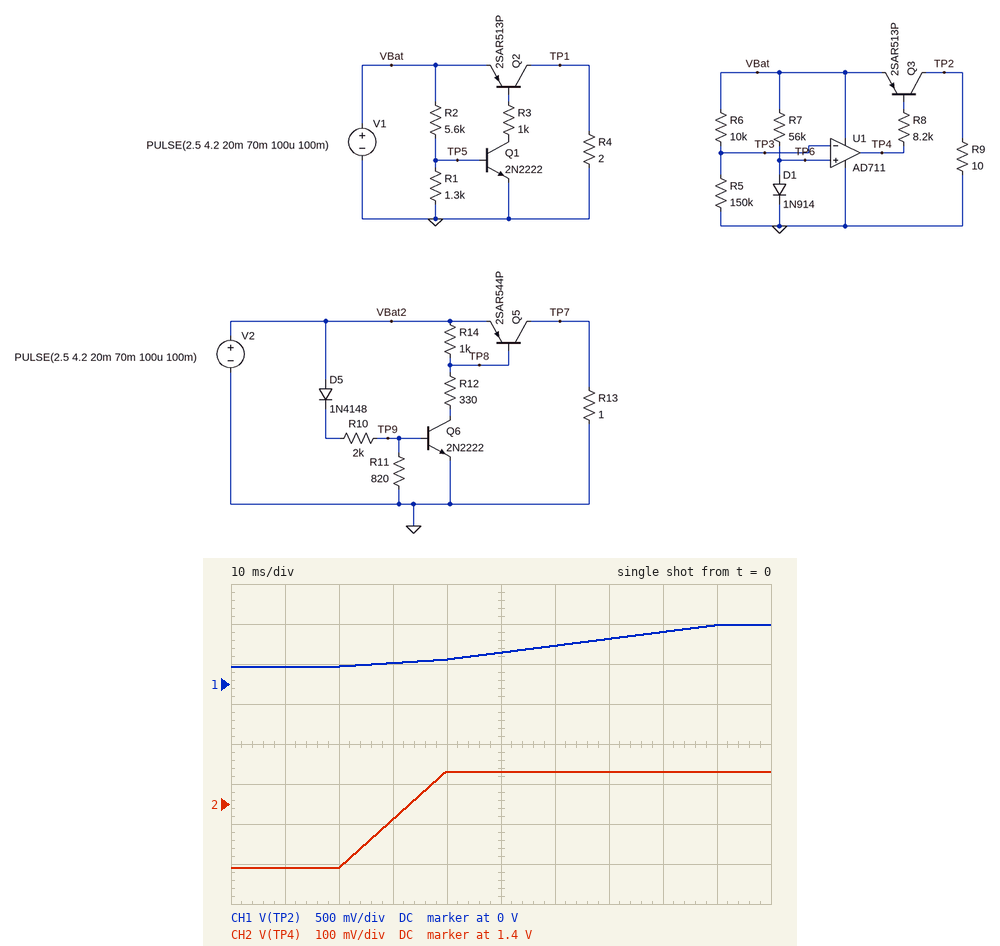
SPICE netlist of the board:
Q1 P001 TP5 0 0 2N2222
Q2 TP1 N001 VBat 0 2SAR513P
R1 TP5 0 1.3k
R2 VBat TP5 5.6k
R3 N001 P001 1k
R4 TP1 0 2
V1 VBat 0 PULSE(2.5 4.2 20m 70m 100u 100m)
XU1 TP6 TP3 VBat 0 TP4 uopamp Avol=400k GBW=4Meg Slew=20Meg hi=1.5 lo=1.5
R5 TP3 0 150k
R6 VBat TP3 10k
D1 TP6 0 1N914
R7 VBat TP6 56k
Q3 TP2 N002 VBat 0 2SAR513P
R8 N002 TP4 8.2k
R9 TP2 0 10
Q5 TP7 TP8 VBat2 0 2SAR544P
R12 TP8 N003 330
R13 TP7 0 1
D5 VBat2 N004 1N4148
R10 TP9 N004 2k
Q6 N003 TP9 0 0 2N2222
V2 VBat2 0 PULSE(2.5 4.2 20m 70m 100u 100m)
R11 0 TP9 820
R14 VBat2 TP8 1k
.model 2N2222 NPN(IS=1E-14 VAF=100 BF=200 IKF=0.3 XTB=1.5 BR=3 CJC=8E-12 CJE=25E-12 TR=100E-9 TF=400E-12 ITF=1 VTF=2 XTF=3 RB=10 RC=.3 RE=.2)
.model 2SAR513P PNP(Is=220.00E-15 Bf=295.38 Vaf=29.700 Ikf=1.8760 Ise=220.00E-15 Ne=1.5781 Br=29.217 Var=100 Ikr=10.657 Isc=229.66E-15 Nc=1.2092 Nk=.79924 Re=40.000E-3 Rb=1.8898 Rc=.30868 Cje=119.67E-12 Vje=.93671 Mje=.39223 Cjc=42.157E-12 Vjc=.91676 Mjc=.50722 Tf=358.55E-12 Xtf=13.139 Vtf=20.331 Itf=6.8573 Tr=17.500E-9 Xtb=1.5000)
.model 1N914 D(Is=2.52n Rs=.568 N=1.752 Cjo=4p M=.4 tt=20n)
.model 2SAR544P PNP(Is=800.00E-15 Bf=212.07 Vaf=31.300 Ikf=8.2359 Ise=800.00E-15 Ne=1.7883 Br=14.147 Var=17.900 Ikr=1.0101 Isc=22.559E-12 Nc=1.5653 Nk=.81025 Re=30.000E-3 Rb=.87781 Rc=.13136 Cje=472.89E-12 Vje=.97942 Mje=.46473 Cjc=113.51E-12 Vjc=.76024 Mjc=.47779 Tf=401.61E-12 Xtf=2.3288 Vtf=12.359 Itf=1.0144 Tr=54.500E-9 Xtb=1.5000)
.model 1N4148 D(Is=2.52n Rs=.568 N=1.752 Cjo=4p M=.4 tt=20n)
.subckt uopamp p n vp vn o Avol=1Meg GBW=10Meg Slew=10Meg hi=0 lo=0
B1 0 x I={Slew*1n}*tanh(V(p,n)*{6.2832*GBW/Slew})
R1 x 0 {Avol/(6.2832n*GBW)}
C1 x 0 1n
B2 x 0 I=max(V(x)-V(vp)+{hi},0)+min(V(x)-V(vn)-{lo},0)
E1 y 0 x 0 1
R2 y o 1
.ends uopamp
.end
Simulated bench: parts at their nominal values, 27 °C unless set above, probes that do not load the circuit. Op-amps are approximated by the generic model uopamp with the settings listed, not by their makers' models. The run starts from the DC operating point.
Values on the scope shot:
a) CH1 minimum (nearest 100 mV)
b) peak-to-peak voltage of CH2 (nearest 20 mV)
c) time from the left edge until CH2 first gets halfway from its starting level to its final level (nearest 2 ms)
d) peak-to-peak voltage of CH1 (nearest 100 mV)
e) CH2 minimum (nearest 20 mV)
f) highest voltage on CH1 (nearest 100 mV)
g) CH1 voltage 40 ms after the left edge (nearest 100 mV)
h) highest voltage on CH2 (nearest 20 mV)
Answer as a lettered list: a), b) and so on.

a) 200 mV
b) 240 mV
c) 30 ms
d) 500 mV
e) 1.24 V
f) 700 mV
g) 300 mV
h) 1.48 V
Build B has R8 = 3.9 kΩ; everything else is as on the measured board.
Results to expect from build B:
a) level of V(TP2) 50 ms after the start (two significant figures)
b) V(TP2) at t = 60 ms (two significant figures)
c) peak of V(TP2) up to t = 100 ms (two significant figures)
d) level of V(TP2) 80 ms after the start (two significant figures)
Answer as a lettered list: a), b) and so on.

a) 780 mV
b) 940 mV
c) 1.4 V
d) 1.3 V
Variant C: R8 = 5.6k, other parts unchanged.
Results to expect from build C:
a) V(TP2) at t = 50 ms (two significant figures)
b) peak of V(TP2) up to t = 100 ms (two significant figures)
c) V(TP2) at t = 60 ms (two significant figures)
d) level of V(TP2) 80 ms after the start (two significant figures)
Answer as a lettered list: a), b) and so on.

a) 560 mV
b) 1.0 V
c) 680 mV
d) 920 mV
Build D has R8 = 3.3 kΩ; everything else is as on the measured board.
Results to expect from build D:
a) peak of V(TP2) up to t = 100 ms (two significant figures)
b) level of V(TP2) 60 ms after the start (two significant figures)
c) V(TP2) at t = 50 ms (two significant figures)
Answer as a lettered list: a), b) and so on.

a) 1.6 V
b) 1.1 V
c) 900 mV
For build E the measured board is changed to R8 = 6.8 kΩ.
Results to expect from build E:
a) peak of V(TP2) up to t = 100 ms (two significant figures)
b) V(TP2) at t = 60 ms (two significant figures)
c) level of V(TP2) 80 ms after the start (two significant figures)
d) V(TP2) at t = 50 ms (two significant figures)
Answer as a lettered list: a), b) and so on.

a) 870 mV
b) 570 mV
c) 770 mV
d) 470 mV
